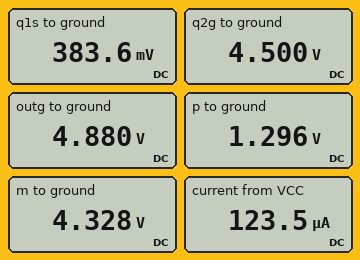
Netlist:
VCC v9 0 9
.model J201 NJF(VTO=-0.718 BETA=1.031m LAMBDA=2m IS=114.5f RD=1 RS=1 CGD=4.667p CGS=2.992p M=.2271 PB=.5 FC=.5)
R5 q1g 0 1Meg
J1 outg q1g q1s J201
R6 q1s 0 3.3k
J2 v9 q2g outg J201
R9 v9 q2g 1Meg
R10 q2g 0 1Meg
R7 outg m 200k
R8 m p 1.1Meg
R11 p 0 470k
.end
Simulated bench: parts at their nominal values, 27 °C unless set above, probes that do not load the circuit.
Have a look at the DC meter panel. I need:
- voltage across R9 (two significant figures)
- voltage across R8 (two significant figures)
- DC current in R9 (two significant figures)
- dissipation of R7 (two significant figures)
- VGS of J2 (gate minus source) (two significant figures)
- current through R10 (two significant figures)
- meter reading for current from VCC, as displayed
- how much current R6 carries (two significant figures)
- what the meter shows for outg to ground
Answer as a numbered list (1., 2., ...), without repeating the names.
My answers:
1. 4.5 V
2. 3.0 V
3. 4.5 µA
4. 1.5 µW
5. -380 mV
6. 4.5 µA
7. 123.5 µA
8. 120 µA
9. 4.880 V
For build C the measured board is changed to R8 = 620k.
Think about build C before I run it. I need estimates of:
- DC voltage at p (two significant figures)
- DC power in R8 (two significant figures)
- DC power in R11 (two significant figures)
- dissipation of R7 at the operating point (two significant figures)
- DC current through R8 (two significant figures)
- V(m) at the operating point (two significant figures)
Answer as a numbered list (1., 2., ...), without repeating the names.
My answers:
1. 1.8 V
2. 8.9 µW
3. 6.7 µW
4. 2.9 µW
5. 3.8 µA
6. 4.1 V
